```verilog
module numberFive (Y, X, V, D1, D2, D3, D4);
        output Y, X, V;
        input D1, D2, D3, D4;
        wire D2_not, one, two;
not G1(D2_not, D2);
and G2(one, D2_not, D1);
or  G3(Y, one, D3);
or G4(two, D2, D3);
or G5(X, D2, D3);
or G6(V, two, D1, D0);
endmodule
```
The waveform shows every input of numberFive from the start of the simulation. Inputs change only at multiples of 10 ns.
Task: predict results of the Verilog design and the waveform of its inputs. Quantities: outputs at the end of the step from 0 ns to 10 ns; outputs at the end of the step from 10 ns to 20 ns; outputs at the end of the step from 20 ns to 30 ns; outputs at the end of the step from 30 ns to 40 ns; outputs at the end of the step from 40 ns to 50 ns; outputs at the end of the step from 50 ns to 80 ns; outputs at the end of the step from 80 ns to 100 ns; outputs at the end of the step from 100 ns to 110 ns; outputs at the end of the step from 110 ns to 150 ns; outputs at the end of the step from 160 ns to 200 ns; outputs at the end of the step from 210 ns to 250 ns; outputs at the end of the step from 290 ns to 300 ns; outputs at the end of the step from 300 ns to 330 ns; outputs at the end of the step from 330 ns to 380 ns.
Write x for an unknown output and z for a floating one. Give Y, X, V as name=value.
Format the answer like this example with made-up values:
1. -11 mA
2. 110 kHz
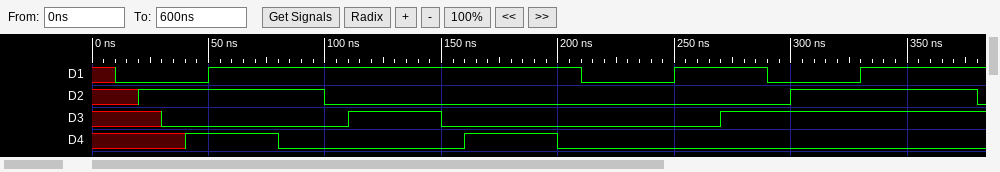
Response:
1. Y=x, X=x, V=x
2. Y=x, X=x, V=x
3. Y=x, X=1, V=1
4. Y=0, X=1, V=1
5. Y=0, X=1, V=1
6. Y=0, X=1, V=1
7. Y=0, X=1, V=1
8. Y=1, X=0, V=1
9. Y=1, X=1, V=1
10. Y=1, X=0, V=1
11. Y=0, X=0, V=x
12. Y=1, X=1, V=1
13. Y=1, X=1, V=1
14. Y=1, X=1, V=1
